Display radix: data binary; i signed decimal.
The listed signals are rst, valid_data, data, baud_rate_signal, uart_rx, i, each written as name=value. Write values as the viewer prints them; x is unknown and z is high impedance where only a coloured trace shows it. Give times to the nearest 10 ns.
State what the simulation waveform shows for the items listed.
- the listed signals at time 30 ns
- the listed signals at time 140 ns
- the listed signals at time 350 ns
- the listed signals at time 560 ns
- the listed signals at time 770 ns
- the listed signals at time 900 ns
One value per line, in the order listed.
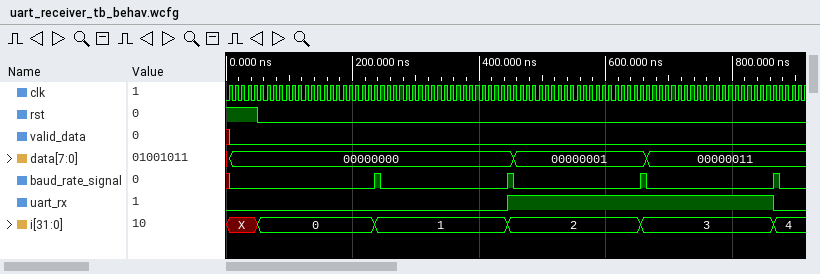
rst=1, valid_data=0, data=00000000, baud_rate_signal=0, uart_rx=0, i=X
rst=0, valid_data=0, data=00000000, baud_rate_signal=0, uart_rx=0, i=0
rst=0, valid_data=0, data=00000000, baud_rate_signal=0, uart_rx=0, i=1
rst=0, valid_data=0, data=00000001, baud_rate_signal=0, uart_rx=1, i=2
rst=0, valid_data=0, data=00000011, baud_rate_signal=0, uart_rx=1, i=3
rst=0, valid_data=0, data=00000011, baud_rate_signal=0, uart_rx=0, i=4
